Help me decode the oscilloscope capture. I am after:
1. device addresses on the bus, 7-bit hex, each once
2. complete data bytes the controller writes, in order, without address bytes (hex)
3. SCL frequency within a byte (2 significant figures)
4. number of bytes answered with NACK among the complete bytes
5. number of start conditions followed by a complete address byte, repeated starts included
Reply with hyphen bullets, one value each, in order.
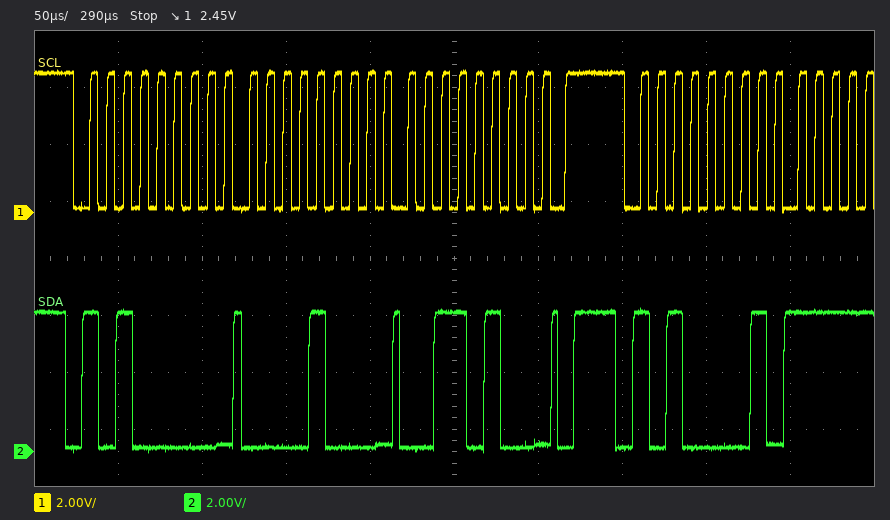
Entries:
- 0x50
- 08 34
- 100 kHz
- 0
- 2
